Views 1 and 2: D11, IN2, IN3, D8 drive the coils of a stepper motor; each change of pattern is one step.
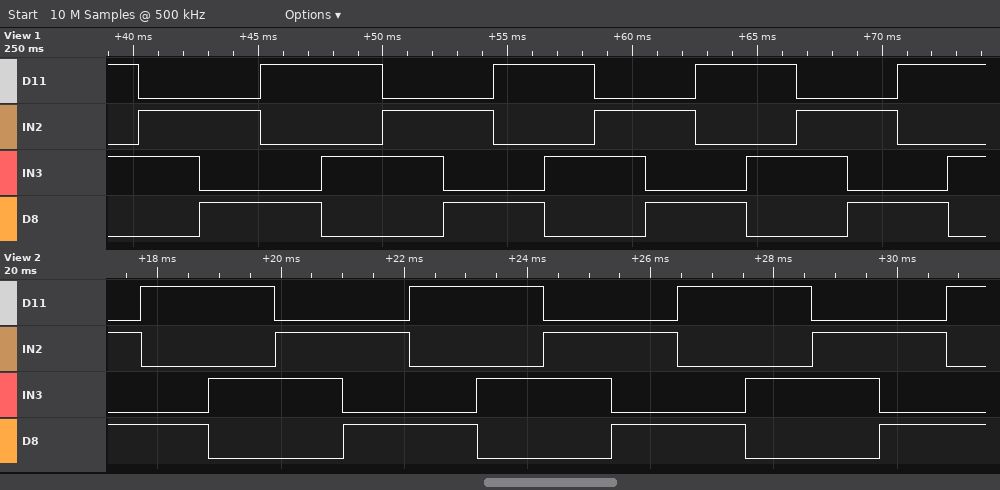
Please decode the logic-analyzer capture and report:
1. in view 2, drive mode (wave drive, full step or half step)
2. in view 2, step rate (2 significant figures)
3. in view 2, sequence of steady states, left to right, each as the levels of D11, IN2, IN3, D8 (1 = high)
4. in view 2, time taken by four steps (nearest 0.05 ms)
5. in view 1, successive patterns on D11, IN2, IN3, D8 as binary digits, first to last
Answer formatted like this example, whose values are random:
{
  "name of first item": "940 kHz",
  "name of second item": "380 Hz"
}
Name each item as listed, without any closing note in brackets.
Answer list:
{
  "in view 2, drive mode": "full step",
  "in view 2, step rate": "920 steps/s",
  "in view 2, sequence of steady states, left to right, each as the levels of D11, IN2, IN3, D8": "0101 1001 1010 0110 0101 1001 1010 0110 0101 1001 1010 0110 0101 1001",
  "in view 2, time taken by four steps": "4.35 ms",
  "in view 1, successive patterns on D11, IN2, IN3, D8 as binary digits, first to last": "1010 0110 0101 1001 1010 0110 0101 1001 1010 0110 0101 1001 1010 0110 0101 1001 1010"
}
